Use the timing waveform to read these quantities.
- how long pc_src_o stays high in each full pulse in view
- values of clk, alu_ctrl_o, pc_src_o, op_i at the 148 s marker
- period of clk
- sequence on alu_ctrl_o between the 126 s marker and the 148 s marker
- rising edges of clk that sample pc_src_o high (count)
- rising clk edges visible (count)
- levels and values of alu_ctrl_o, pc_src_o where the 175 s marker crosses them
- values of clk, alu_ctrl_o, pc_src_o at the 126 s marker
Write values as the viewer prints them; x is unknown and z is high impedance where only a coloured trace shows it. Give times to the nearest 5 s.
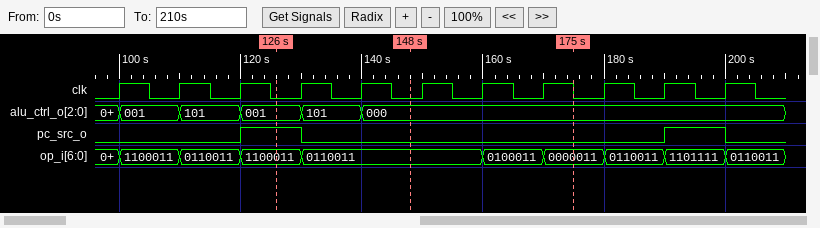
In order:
10 s, 10 s
clk=0, alu_ctrl_o=000, pc_src_o=0, op_i=0110011
10 s
001, 101, 000
2
11
alu_ctrl_o=000, pc_src_o=0
clk=0, alu_ctrl_o=001, pc_src_o=1
